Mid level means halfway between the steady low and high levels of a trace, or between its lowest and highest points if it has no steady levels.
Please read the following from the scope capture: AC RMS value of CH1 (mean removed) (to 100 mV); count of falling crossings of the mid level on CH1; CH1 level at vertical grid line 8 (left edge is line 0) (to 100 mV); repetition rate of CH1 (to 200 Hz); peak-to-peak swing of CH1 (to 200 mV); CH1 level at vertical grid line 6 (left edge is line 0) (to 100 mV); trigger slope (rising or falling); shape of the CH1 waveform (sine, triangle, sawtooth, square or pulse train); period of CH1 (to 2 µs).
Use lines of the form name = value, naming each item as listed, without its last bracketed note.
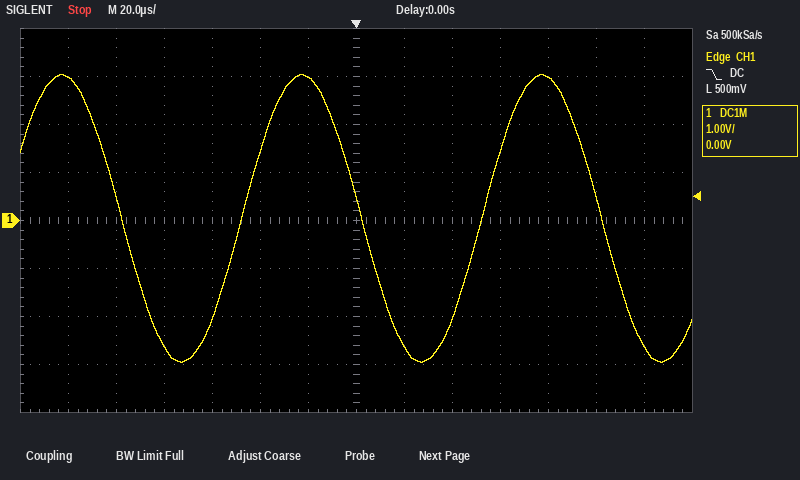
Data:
AC RMS value of CH1 (mean removed) = 2.1 V
count of falling crossings of the mid level on CH1 = 3
CH1 level at vertical grid line 8 (left edge is line 0) = -2.6 V
repetition rate of CH1 = 10.0 kHz
peak-to-peak swing of CH1 = 6.0 V
CH1 level at vertical grid line 6 (left edge is line 0) = 3.0 V
trigger slope = falling
shape of the CH1 waveform = sine
period of CH1 = 100 µs
